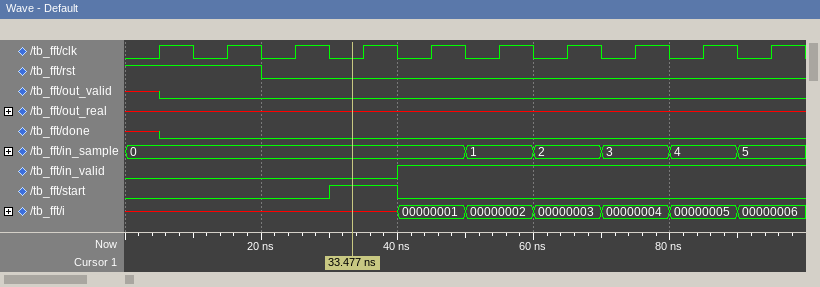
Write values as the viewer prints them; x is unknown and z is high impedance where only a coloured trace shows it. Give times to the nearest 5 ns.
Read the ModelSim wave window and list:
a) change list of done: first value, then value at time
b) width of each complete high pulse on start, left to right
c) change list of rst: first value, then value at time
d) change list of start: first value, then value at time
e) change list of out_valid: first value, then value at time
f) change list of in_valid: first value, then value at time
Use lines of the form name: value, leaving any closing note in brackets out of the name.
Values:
change list of done: first value, then value at time: x, 0 at 5 ns
width of each complete high pulse on start, left to right: 10 ns
change list of rst: first value, then value at time: 1, 0 at 20 ns
change list of start: first value, then value at time: 0, 1 at 30 ns, 0 at 40 ns
change list of out_valid: first value, then value at time: x, 0 at 5 ns
change list of in_valid: first value, then value at time: 0, 1 at 40 ns
